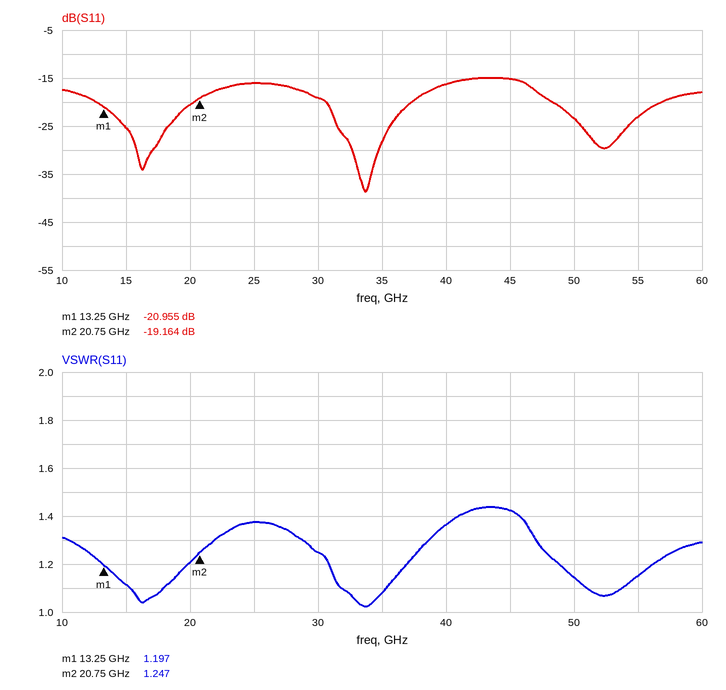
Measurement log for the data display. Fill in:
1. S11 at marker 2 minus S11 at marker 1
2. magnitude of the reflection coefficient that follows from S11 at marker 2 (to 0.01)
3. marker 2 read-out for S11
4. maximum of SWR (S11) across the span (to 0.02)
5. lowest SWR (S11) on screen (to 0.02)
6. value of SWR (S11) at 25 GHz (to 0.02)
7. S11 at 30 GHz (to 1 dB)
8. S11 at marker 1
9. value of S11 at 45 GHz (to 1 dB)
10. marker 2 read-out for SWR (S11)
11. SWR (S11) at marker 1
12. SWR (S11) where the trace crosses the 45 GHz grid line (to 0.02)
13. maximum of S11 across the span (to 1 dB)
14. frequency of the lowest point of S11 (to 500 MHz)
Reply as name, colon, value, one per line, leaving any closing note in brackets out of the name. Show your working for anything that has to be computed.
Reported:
S11 at marker 2 minus S11 at marker 1: -19.164 − (-20.955) = 1.791 dB
magnitude of the reflection coefficient that follows from S11 at marker 2: 10^(-19.164/20) ≈ 0.11
marker 2 read-out for S11: -19.164 dB
maximum of SWR (S11) across the span: 1.44
lowest SWR (S11) on screen: 1.02
value of SWR (S11) at 25 GHz: 1.38
S11 at 30 GHz: -19 dB
S11 at marker 1: -20.955 dB
value of S11 at 45 GHz: -15 dB
marker 2 read-out for SWR: 1.247
SWR (S11) at marker 1: 1.197
SWR (S11) where the trace crosses the 45 GHz grid line: 1.42
maximum of S11 across the span: -15 dB
frequency of the lowest point of S11: 33.5 GHz
